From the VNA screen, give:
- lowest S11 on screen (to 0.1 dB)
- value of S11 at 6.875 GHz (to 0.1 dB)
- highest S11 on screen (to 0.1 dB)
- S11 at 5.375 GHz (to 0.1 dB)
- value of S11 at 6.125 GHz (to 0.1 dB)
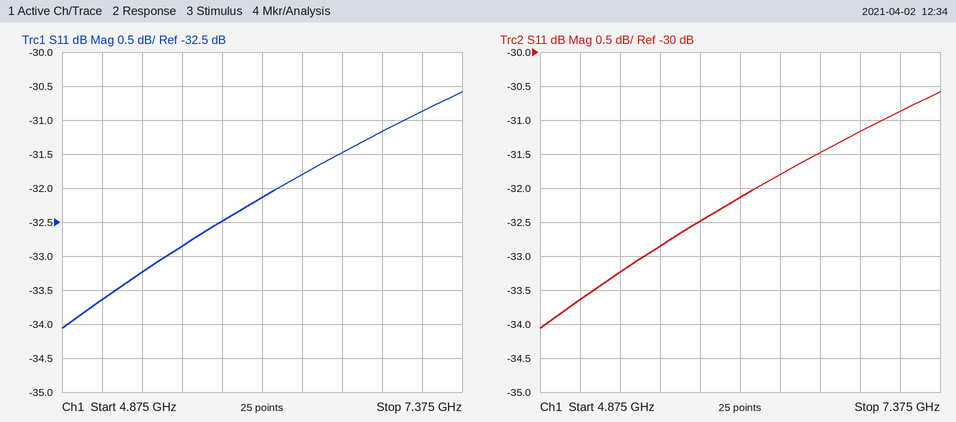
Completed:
-34.1 dB
-31.2 dB
-30.6 dB
-33.2 dB
-32.1 dB
